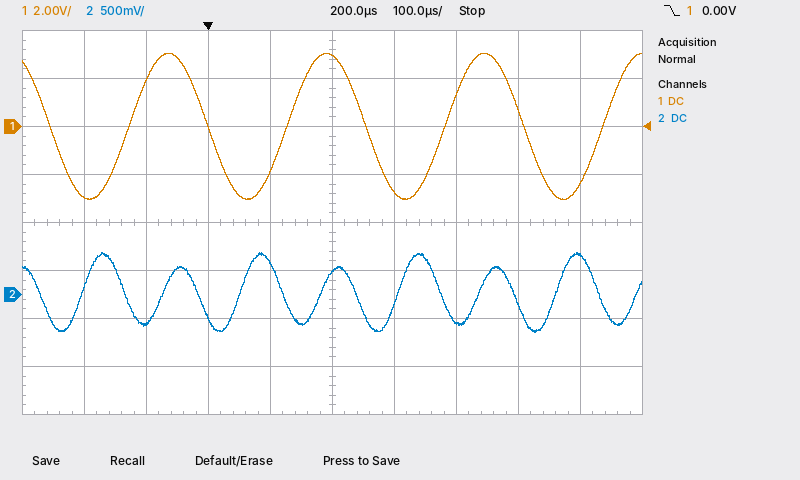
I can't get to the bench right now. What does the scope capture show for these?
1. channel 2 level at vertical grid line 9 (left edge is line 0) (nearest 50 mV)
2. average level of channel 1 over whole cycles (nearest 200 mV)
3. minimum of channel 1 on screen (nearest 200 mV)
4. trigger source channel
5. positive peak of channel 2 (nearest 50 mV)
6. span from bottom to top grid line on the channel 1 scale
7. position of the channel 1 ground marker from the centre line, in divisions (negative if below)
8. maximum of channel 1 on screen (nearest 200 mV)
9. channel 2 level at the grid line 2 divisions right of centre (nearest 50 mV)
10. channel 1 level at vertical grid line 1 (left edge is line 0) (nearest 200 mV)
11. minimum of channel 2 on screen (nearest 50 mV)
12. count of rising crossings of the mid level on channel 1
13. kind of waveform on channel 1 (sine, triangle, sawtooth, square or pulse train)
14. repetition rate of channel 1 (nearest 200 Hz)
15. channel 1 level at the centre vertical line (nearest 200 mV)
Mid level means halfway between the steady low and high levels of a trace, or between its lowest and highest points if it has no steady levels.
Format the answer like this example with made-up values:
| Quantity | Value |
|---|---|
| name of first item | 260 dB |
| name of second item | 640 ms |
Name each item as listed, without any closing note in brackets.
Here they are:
| Quantity | Value |
|---|---|
| channel 2 level at vertical grid line 9 (left edge is line 0) | 400 mV |
| average level of channel 1 over whole cycles | 0.0 V |
| minimum of channel 1 on screen | -3.0 V |
| trigger source channel | channel 1 |
| positive peak of channel 2 | 450 mV |
| span from bottom to top grid line on the channel 1 scale | 16 V |
| position of the channel 1 ground marker from the centre line, in divisions | +2.0 div |
| maximum of channel 1 on screen | 3.0 V |
| channel 2 level at the grid line 2 divisions right of centre | -300 mV |
| channel 1 level at vertical grid line 1 (left edge is line 0) | -3.0 V |
| minimum of channel 2 on screen | -400 mV |
| count of rising crossings of the mid level on channel 1 | 4 |
| kind of waveform on channel 1 | sine |
| repetition rate of channel 1 | 4.0 kHz |
| channel 1 level at the centre vertical line | 3.0 V |
